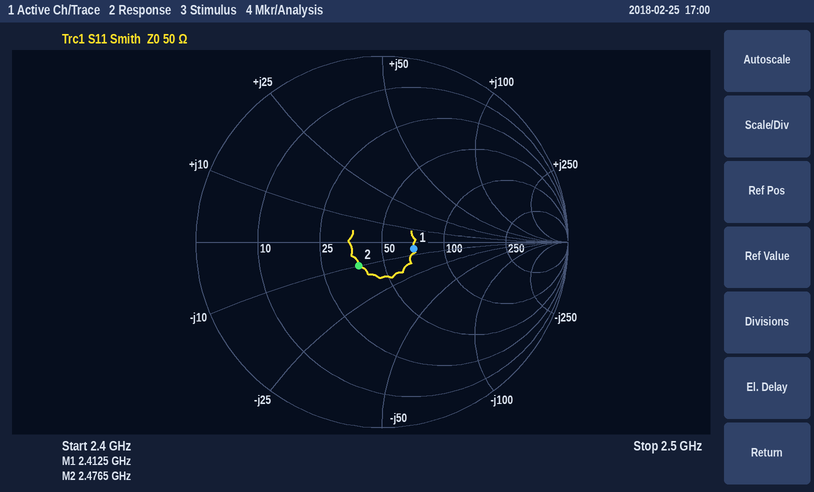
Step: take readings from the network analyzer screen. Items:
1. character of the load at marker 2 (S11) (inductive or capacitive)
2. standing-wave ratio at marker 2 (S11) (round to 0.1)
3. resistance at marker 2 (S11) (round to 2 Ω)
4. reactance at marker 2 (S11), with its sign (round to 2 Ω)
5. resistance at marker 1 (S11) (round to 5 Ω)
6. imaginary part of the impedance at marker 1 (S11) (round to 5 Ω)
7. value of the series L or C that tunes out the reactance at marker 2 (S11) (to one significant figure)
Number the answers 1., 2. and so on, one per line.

1. capacitive
2. 1.4
3. 38 Ω
4. -10 Ω
5. 70 Ω
6. -5 Ω
7. 600 pH
